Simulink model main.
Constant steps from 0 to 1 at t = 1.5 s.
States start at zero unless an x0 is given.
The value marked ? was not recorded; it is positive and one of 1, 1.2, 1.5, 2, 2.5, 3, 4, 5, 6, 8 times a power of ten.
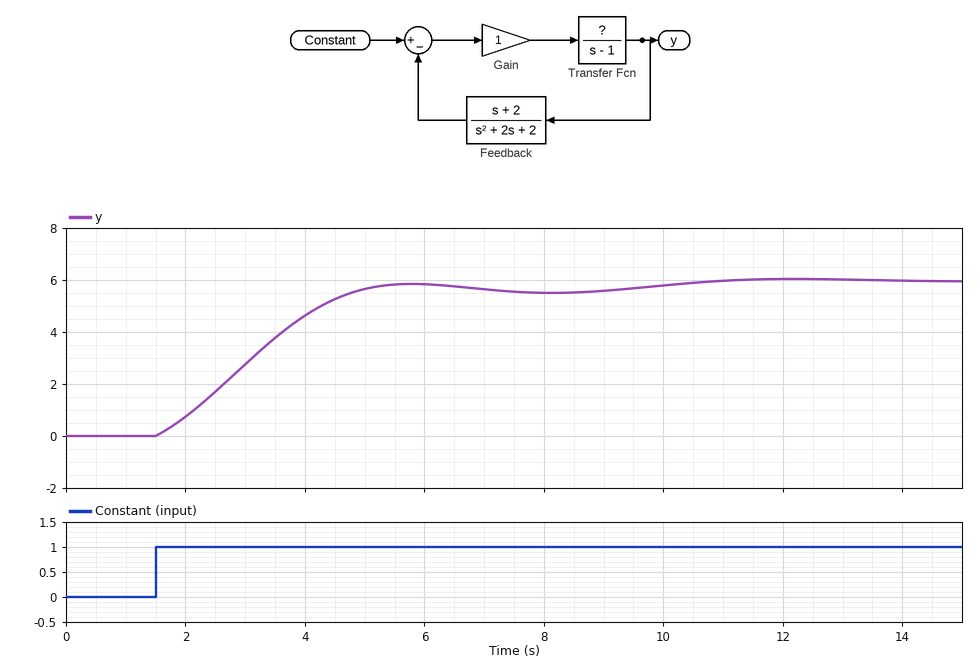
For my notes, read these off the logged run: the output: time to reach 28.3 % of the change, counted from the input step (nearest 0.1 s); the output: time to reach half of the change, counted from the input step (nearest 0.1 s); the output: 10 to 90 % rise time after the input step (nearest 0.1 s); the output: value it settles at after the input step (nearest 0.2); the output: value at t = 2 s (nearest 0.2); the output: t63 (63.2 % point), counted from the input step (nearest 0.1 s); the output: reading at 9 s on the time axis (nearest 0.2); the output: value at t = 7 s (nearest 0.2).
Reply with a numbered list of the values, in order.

1. 1.0 s
2. 1.6 s
3. 2.7 s
4. 6.0
5. 0.8
6. 2.0 s
7. 5.6
8. 5.6
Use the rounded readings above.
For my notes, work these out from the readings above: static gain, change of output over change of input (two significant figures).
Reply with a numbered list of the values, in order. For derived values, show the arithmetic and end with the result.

1. (6 - 0) / (1 - 0) = 6.0
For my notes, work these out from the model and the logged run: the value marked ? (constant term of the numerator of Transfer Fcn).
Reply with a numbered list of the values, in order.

1. 1.2
